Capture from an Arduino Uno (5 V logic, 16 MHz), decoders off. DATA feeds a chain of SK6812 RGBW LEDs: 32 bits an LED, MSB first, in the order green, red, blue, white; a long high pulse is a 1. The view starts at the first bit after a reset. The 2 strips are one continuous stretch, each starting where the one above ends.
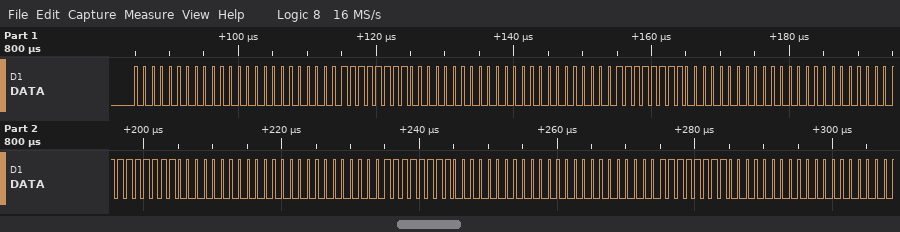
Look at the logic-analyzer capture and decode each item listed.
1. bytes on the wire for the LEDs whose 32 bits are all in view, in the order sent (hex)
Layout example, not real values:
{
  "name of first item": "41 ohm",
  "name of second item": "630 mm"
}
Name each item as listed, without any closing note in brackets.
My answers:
{
  "bytes on the wire for the LEDs whose 32 bits are all in view, in the order sent": "00 00 00 FF 00 00 00 FF 00 00 00 FF 00 00 00 FF 00 00 00 FF"
}
